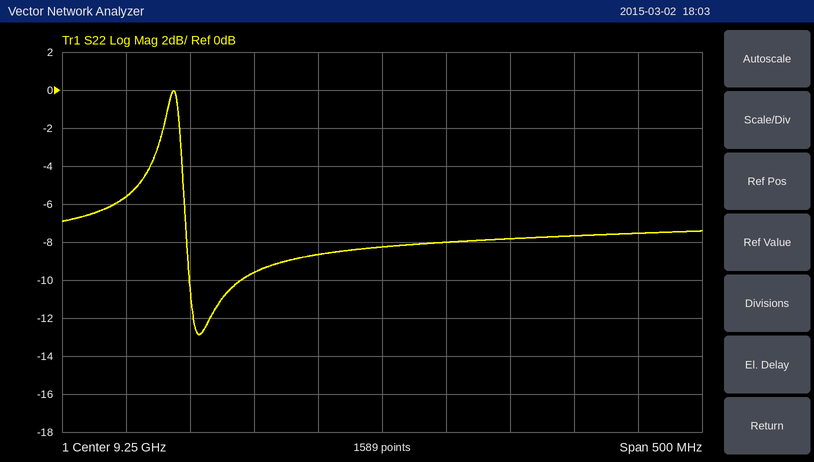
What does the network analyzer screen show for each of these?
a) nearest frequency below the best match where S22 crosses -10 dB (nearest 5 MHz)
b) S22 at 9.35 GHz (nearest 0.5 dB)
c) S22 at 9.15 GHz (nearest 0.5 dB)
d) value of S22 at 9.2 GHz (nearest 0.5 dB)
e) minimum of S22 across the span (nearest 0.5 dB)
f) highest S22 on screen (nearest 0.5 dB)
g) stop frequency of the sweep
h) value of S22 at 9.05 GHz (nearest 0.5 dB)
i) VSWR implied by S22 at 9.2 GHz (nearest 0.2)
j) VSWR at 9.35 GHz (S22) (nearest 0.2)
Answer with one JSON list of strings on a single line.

["9.100 GHz", "-8.0 dB", "-9.5 dB", "-8.5 dB", "-13.0 dB", "0.0 dB", "9.5 GHz", "-5.5 dB", "2.2", "2.4"]
